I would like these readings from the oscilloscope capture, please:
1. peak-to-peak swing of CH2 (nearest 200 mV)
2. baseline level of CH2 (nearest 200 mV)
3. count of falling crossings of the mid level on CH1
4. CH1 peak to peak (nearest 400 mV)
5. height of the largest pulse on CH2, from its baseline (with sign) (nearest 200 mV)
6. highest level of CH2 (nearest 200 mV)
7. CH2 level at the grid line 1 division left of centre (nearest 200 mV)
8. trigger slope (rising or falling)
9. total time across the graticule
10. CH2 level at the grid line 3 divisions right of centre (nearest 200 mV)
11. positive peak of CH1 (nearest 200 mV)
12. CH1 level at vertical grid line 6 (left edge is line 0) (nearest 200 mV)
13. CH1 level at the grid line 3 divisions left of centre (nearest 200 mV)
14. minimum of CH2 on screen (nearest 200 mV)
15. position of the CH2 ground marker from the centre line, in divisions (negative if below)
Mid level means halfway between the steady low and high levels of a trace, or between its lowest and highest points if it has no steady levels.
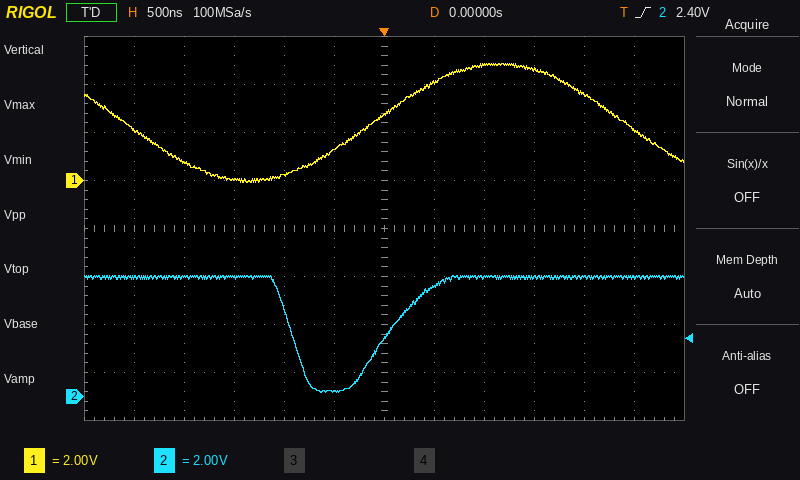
4.8 V
5.0 V
2
4.8 V
-4.8 V
5.0 V
200 mV
rising
6 µs
5.0 V
4.8 V
2.8 V
0.0 V
200 mV
-3.5 div
